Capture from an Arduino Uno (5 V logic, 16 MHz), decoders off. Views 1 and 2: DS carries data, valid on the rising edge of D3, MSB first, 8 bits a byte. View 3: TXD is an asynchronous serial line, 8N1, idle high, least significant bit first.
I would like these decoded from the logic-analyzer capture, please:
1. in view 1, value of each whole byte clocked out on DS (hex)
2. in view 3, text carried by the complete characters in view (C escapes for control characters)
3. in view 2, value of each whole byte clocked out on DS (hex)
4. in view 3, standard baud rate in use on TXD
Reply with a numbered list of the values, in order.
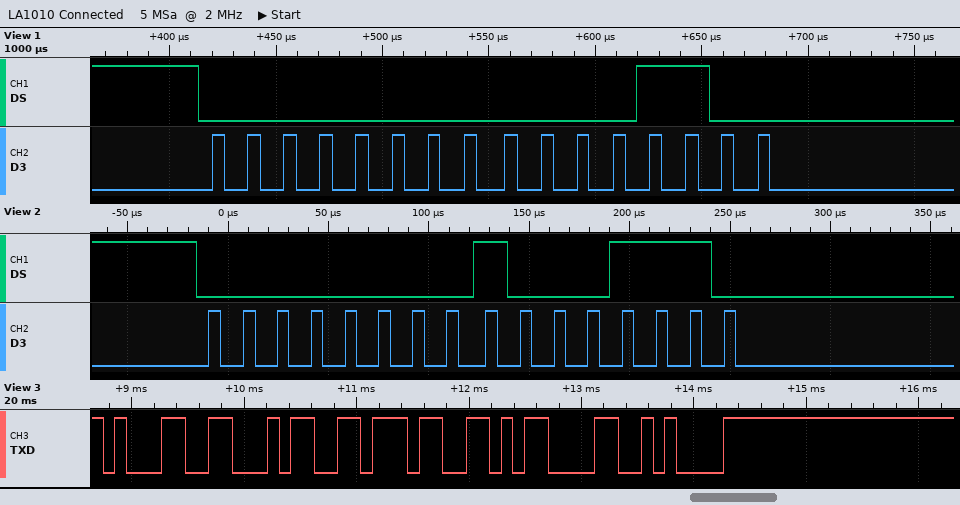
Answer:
1. 0x00 0x0C
2. "147\r\n"
3. 00 8E
4. 9600 baud
